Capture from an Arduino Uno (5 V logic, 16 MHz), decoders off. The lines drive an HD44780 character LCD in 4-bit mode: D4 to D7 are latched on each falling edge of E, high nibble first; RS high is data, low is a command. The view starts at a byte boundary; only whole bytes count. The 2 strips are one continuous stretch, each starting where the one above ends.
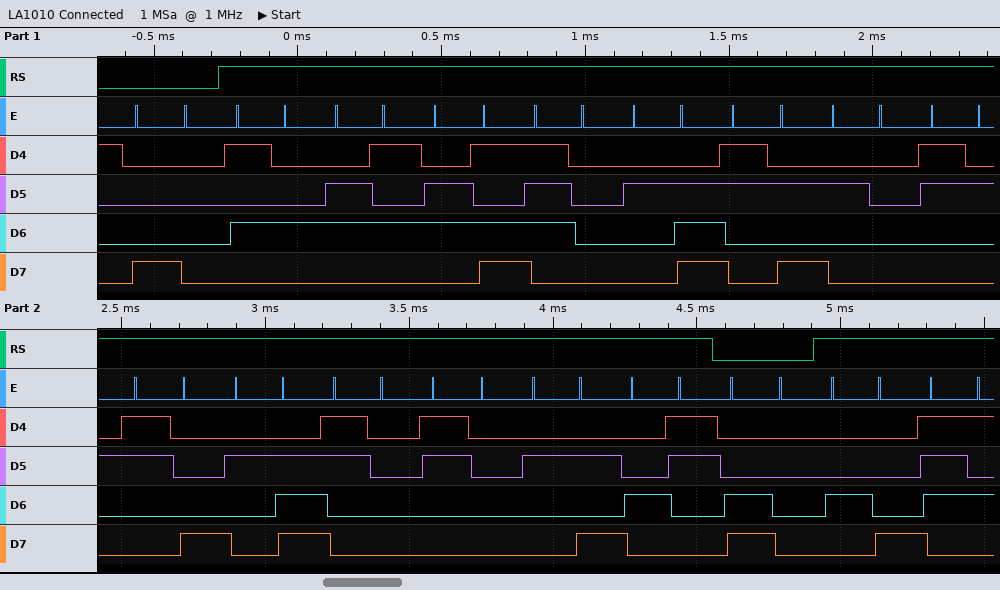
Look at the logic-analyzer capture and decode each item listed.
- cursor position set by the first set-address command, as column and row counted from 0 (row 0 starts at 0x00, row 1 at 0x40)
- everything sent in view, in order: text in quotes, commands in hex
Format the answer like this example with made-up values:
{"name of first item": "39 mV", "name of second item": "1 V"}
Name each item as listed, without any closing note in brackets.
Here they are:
{"cursor position set by the first set-address command, as column and row counted from 0": "column 0, row 0", "everything sent in view, in order: text in quotes, commands in hex": "0x80 \"Temp.: 28.00*C\" 0xC0 \"Hu\""}
